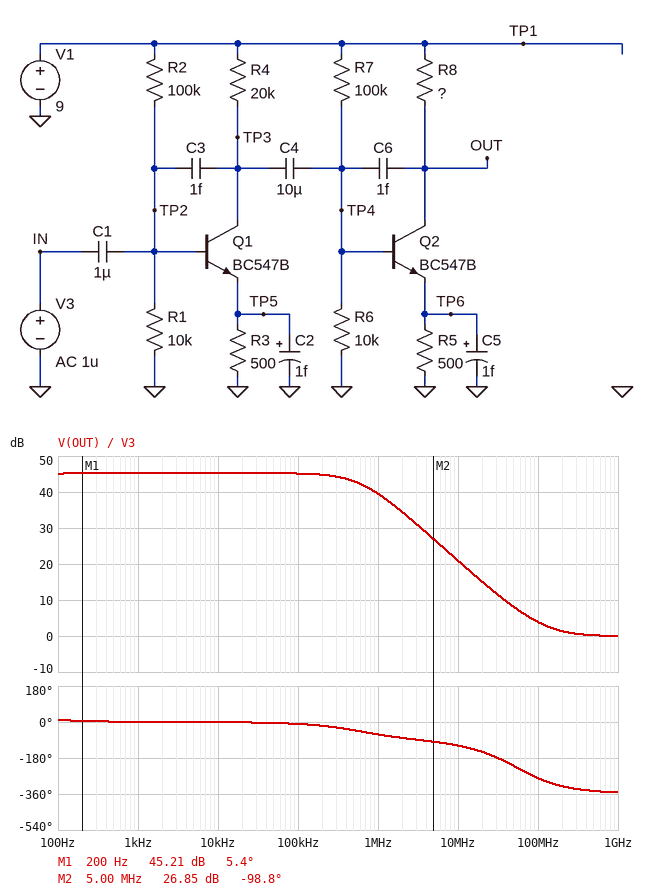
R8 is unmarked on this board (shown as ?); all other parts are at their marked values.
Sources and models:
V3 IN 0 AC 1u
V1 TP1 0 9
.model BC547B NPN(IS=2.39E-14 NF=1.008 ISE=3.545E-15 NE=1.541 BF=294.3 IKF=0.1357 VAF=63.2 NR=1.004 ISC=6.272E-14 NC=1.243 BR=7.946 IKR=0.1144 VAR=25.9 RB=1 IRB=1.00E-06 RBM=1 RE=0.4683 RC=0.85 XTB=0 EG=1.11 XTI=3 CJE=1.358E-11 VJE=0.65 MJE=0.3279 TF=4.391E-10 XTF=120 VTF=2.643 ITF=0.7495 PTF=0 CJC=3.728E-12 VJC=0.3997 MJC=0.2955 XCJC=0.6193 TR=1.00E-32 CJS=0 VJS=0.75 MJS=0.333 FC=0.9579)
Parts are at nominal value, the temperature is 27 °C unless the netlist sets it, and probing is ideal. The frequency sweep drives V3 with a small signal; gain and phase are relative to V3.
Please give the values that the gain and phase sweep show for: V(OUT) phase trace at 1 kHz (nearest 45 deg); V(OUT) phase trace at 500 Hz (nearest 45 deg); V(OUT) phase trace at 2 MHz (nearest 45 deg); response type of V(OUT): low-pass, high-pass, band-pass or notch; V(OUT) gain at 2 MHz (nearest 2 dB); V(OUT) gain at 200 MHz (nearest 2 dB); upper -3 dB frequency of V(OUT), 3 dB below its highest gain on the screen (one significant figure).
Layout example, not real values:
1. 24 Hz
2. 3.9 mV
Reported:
1. 0 deg
2. 0 deg
3. -90 deg
4. low-pass
5. 34 dB
6. 2 dB
7. 600 kHz
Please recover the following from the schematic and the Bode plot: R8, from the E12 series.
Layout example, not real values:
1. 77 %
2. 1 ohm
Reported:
1. 10 kΩ
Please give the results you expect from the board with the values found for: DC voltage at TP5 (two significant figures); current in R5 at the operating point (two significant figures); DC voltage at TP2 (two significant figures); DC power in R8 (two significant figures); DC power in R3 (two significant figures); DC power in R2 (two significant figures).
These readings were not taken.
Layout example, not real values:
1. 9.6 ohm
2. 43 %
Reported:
1. 190 mV
2. 390 µA
3. 810 mV
4. 1.5 mW
5. 74 µW
6. 670 µW
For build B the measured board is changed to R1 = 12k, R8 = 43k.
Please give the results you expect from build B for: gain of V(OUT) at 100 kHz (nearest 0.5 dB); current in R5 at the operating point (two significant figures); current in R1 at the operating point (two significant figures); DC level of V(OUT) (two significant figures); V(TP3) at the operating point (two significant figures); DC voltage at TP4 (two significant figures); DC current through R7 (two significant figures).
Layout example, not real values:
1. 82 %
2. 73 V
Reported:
1. -0.5 dB
2. 220 µA
3. 70 µA
4. 150 mV
5. 280 mV
6. 710 mV
7. 83 µA
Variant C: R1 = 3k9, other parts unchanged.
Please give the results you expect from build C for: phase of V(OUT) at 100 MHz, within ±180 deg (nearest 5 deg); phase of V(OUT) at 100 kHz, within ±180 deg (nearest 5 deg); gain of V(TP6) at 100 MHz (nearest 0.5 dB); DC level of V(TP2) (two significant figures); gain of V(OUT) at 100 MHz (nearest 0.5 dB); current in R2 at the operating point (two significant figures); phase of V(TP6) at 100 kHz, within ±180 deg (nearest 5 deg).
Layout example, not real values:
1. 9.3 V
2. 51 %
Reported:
1. 85 deg
2. -75 deg
3. -9.0 dB
4. 340 mV
5. -3.5 dB
6. 87 µA
7. 105 deg
